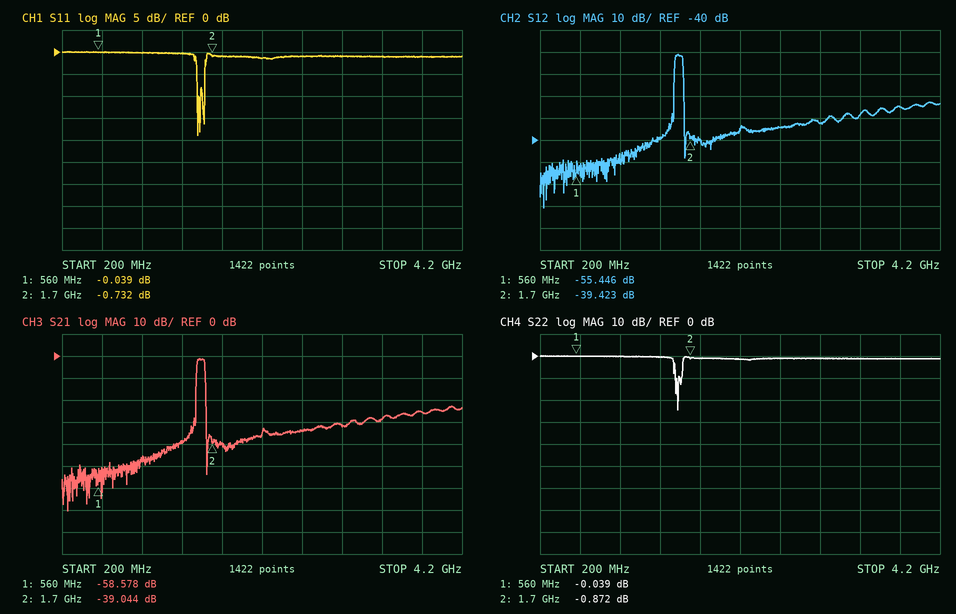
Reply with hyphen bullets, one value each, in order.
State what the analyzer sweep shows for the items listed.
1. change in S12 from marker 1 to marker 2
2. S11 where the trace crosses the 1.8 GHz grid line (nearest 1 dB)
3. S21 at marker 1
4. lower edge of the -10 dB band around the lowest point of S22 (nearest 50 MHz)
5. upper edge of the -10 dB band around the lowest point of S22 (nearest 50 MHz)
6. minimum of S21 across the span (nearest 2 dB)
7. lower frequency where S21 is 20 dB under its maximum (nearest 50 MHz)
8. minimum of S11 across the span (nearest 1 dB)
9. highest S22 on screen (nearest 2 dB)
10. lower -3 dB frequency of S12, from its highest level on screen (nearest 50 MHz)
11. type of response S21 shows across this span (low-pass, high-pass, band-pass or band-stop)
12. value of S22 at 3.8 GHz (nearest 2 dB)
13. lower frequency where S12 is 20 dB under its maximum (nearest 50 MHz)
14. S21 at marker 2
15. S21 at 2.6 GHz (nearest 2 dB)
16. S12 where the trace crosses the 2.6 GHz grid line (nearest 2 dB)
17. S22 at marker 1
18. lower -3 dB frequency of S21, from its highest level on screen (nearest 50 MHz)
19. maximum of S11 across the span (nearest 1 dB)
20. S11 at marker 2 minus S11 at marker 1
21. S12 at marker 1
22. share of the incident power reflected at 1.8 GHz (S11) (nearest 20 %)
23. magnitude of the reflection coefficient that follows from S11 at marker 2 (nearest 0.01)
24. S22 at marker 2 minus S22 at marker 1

- 16.023 dB
- -1 dB
- -58.578 dB
- 1.55 GHz
- 1.60 GHz
- -70 dB
- 1.55 GHz
- -19 dB
- 0 dB
- 1.55 GHz
- band-pass
- -2 dB
- 1.55 GHz
- -39.044 dB
- -34 dB
- -34 dB
- -0.039 dB
- 1.55 GHz
- 0 dB
- -0.693 dB
- -55.446 dB
- 80 %
- 0.92
- -0.833 dB
